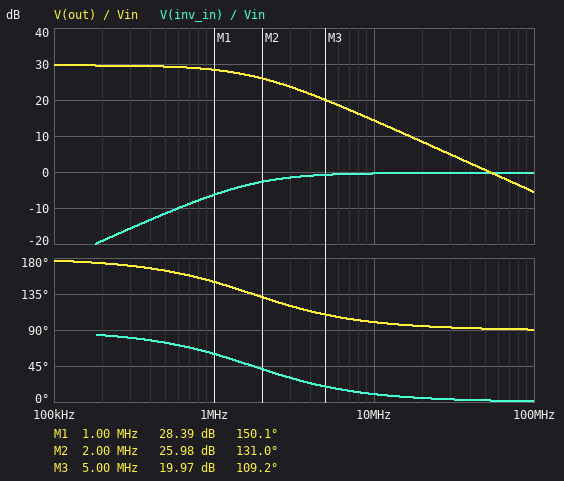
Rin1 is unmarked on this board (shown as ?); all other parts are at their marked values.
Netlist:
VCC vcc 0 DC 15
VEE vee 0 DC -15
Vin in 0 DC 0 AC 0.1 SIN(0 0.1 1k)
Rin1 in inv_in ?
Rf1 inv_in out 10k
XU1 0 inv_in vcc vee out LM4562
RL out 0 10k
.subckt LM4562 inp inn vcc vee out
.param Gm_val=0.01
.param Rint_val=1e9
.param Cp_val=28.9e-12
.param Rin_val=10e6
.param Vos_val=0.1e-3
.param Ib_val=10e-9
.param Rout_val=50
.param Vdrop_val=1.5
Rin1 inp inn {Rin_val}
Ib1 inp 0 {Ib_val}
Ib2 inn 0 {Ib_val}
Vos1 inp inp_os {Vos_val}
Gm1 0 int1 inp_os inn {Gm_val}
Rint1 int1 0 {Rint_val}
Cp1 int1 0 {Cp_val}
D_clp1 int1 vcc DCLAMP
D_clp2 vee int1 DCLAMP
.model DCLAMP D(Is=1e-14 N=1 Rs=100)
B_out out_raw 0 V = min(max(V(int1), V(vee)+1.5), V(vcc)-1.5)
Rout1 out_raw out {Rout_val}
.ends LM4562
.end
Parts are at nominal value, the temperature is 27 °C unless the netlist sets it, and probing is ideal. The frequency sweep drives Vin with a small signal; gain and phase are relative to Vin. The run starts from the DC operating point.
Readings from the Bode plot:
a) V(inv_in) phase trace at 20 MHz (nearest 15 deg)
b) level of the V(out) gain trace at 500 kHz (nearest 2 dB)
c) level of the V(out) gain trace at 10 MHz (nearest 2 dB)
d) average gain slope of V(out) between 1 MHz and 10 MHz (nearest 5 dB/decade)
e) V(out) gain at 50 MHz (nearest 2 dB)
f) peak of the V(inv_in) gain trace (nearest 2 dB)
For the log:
0 deg
30 dB
14 dB
-15 dB/decade
0 dB
0 dB
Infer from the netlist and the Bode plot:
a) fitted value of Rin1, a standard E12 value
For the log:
330 Ω
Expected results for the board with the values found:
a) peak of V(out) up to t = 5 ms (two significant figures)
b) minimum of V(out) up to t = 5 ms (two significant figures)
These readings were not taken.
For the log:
3.0 V
-3.0 V
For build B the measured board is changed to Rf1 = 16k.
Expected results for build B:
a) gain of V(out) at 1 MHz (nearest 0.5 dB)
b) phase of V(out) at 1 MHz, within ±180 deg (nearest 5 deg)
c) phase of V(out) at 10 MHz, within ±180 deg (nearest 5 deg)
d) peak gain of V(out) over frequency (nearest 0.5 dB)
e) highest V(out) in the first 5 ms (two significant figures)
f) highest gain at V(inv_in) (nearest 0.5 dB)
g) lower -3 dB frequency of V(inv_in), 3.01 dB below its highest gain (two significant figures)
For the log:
31.0 dB
140 deg
95 deg
33.5 dB
4.8 V
0 dB
1.1 MHz
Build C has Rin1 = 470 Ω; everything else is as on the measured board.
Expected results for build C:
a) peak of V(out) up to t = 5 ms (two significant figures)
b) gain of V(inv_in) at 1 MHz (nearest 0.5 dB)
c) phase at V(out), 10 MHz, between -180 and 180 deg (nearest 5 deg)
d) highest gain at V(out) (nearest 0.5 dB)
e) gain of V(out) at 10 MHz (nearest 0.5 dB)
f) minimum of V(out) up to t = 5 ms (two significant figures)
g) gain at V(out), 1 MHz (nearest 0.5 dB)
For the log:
2.1 V
-9.0 dB
105 deg
26.5 dB
14.0 dB
-2.1 V
26.0 dB
